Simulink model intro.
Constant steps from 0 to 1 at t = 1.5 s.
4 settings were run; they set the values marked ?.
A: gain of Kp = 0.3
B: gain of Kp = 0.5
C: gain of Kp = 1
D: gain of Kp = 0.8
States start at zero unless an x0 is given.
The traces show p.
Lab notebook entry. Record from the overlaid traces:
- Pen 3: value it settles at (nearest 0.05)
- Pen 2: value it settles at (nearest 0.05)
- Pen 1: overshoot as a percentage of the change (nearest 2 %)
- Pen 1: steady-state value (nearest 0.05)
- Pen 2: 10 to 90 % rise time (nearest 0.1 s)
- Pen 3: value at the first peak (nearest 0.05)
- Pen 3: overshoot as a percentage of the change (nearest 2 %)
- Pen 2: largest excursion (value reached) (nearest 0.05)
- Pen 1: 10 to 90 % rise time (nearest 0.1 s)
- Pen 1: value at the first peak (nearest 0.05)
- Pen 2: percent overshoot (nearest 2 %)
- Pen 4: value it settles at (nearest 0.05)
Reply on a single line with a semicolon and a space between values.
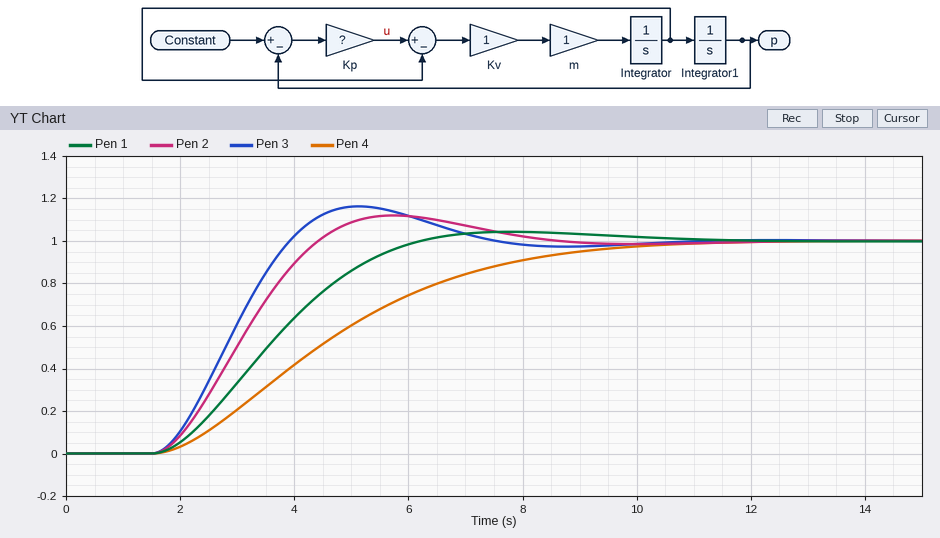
1.00; 1.00; 4 %; 1.00; 2.0 s; 1.15; 16 %; 1.10; 3.0 s; 1.05; 12 %; 1.00
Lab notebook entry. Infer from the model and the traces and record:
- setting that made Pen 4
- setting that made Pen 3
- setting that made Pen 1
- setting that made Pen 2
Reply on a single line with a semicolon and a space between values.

A; C; B; D
